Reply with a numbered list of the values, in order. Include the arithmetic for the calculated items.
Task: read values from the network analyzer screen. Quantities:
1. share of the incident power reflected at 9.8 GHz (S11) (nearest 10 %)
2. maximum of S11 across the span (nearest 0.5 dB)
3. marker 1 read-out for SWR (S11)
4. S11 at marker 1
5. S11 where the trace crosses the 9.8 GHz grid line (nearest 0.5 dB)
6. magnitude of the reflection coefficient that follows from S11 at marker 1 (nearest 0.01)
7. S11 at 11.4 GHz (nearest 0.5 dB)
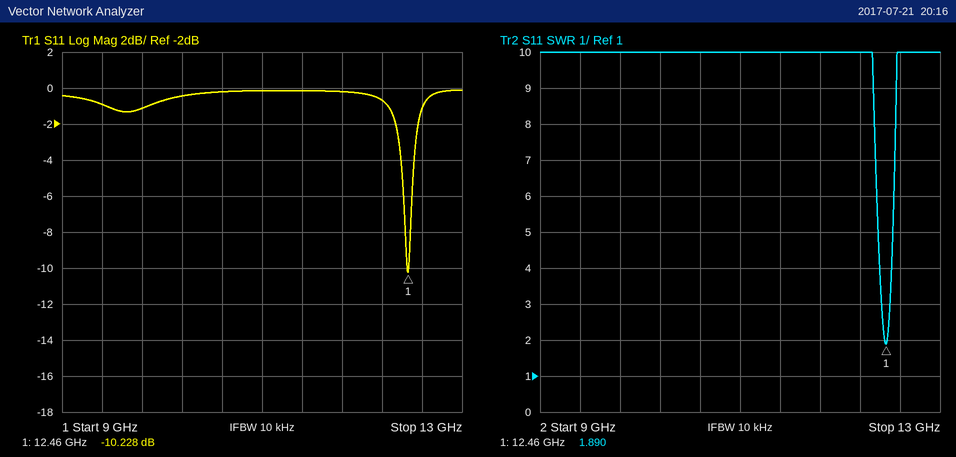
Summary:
1. 10^(-1/10) ≈ 79.4 %, so 80 % to the nearest 10 %
2. 0.0 dB
3. 1.890
4. -10.228 dB
5. -1.0 dB
6. 10^(-10.228/20) ≈ 0.31
7. 0.0 dB
